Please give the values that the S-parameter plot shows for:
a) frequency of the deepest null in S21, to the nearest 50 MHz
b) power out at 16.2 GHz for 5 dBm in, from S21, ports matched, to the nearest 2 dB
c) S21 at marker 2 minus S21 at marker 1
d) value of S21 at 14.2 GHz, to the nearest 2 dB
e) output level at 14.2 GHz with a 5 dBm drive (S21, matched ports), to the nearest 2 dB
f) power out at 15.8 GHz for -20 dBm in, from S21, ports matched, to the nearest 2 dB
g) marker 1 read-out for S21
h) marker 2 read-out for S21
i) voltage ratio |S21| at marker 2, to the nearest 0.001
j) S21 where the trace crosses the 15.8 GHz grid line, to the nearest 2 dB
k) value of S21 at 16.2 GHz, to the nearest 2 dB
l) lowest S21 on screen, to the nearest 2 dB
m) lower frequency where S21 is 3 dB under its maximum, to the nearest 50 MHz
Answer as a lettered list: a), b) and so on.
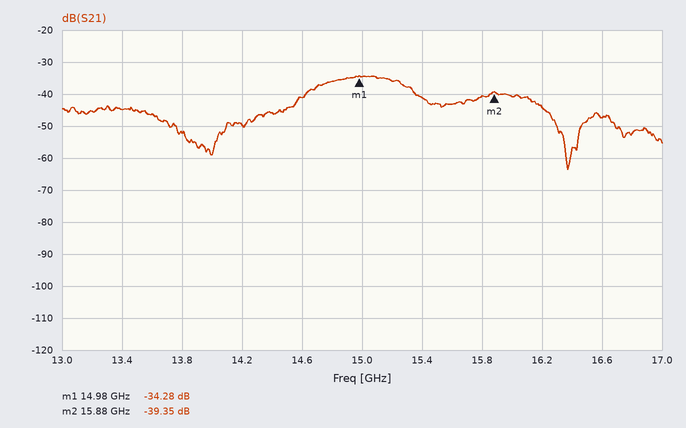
a) 16.35 GHz
b) -40 dBm
c) -5.07 dB
d) -50 dB
e) -44 dBm
f) -60 dBm
g) -34.28 dB
h) -39.35 dB
i) 0.011
j) -40 dB
k) -44 dB
l) -64 dB
m) 14.70 GHz
